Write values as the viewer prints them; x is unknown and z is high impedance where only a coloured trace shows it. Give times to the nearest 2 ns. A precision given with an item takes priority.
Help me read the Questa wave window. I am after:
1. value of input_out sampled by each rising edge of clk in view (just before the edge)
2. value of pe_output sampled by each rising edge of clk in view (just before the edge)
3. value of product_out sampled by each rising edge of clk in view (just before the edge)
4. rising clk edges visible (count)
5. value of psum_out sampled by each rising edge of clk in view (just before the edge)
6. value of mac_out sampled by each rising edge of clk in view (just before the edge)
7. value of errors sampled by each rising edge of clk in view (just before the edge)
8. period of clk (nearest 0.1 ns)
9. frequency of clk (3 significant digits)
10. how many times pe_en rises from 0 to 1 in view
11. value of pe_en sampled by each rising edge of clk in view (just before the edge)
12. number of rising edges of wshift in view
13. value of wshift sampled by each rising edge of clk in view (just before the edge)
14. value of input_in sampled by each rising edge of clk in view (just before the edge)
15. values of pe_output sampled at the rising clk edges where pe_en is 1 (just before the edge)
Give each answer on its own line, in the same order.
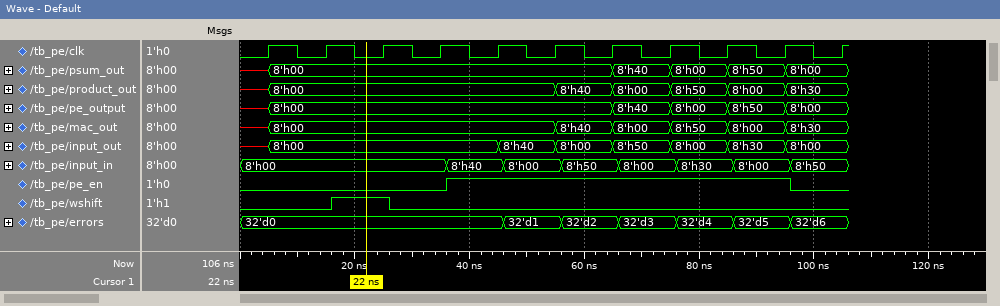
x, 8'h00, 8'h00, 8'h00, 8'h00, 8'h40, 8'h00, 8'h50, 8'h00, 8'h30, 8'h00
x, 8'h00, 8'h00, 8'h00, 8'h00, 8'h00, 8'h00, 8'h40, 8'h00, 8'h50, 8'h00
x, 8'h00, 8'h00, 8'h00, 8'h00, 8'h00, 8'h40, 8'h00, 8'h50, 8'h00, 8'h30
11
x, 8'h00, 8'h00, 8'h00, 8'h00, 8'h00, 8'h00, 8'h40, 8'h00, 8'h50, 8'h00
x, 8'h00, 8'h00, 8'h00, 8'h00, 8'h00, 8'h40, 8'h00, 8'h50, 8'h00, 8'h30
32'd0, 32'd0, 32'd0, 32'd0, 32'd0, 32'd1, 32'd2, 32'd3, 32'd4, 32'd5, 32'd6
10 ns
100 MHz
1
0 0 0 0 1 1 1 1 1 1 0
1
0 0 1 0 0 0 0 0 0 0 0
8'h00, 8'h00, 8'h00, 8'h00, 8'h40, 8'h00, 8'h50, 8'h00, 8'h30, 8'h00, 8'h50
8'h00, 8'h00, 8'h00, 8'h40, 8'h00, 8'h50
